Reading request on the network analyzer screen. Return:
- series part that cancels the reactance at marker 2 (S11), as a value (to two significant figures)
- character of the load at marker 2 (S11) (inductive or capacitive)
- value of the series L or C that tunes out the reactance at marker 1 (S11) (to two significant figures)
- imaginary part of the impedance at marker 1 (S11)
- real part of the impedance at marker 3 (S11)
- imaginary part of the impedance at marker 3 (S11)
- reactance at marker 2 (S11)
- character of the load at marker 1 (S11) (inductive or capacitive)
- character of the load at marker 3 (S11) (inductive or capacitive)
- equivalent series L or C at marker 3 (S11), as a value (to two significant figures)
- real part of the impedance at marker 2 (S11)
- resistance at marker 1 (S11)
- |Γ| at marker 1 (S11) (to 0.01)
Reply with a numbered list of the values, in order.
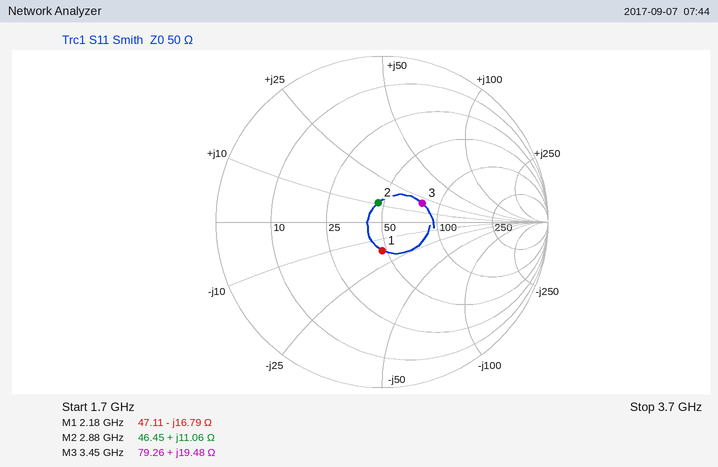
1. 5.0 pF
2. inductive
3. 1.2 nH
4. -16.79 Ω
5. 79.26 Ω
6. +19.48 Ω
7. +11.06 Ω
8. capacitive
9. inductive
10. 900 pH
11. 46.45 Ω
12. 47.11 Ω
13. 0.17
